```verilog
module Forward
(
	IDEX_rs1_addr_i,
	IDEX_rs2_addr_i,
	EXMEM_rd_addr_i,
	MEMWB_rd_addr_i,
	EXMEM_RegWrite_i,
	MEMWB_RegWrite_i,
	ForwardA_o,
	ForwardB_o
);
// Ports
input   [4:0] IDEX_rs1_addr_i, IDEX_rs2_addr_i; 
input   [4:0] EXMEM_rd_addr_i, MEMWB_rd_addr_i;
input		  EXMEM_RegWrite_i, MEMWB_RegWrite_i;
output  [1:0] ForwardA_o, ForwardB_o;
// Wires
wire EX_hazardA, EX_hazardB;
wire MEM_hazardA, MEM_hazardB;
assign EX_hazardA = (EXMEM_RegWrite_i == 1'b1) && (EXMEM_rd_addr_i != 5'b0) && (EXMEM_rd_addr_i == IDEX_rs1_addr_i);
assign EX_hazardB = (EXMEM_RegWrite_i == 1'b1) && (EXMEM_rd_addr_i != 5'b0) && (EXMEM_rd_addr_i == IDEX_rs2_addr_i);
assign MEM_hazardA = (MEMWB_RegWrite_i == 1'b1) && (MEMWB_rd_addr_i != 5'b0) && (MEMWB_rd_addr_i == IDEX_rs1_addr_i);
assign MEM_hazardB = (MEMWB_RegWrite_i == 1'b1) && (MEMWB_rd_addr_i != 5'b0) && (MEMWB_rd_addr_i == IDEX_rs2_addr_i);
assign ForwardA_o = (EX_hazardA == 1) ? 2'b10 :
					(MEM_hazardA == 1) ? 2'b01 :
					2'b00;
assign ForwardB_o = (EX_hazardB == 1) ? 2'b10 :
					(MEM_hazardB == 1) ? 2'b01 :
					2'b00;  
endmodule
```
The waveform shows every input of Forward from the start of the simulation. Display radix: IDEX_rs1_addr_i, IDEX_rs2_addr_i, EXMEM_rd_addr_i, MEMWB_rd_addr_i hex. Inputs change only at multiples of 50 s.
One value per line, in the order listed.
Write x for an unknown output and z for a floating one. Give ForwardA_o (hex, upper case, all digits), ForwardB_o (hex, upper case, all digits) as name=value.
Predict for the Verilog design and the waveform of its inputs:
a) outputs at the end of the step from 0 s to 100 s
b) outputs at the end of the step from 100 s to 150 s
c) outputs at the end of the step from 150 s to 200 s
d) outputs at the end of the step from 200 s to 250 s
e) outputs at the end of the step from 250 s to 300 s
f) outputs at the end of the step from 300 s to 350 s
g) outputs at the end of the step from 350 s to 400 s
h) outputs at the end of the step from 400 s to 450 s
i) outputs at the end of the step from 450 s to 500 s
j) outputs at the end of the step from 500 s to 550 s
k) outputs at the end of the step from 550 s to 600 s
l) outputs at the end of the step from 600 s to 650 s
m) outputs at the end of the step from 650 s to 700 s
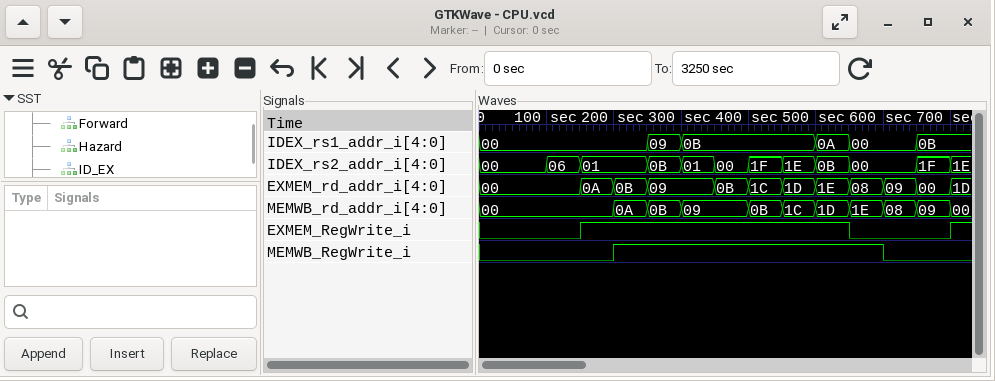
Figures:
ForwardA_o=0, ForwardB_o=0
ForwardA_o=0, ForwardB_o=0
ForwardA_o=0, ForwardB_o=0
ForwardA_o=0, ForwardB_o=0
ForwardA_o=2, ForwardB_o=1
ForwardA_o=0, ForwardB_o=0
ForwardA_o=2, ForwardB_o=0
ForwardA_o=1, ForwardB_o=0
ForwardA_o=0, ForwardB_o=0
ForwardA_o=0, ForwardB_o=0
ForwardA_o=0, ForwardB_o=0
ForwardA_o=0, ForwardB_o=0
ForwardA_o=0, ForwardB_o=0
